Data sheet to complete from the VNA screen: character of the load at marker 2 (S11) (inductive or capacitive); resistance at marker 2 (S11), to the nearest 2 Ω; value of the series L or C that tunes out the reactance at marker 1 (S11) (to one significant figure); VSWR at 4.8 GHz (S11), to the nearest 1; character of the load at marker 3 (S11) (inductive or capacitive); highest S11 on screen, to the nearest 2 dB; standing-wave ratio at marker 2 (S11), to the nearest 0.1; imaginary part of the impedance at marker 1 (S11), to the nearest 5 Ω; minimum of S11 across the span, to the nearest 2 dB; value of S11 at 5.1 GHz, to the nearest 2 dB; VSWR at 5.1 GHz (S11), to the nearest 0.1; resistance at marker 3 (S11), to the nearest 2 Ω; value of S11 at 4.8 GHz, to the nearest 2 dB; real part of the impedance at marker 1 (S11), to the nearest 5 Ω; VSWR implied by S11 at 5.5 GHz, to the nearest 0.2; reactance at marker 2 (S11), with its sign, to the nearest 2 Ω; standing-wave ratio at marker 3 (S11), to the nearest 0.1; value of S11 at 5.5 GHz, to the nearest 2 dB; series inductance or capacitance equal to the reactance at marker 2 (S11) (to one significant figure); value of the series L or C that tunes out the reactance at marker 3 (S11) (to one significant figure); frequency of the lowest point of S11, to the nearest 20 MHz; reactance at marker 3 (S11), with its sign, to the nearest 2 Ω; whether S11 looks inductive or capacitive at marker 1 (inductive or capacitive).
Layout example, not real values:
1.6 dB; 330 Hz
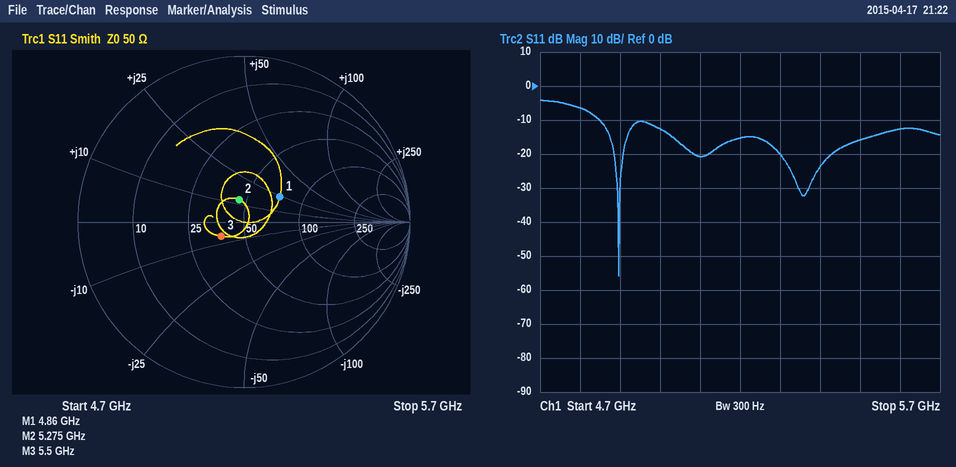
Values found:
inductive; 46 Ω; 1 pF; 3; capacitive; -4 dB; 1.3; +25 Ω; -56 dB; -20 dB; 1.2; 38 Ω; -6 dB; 75 Ω; 1.4; +12 Ω; 1.4; -16 dB; 400 pH; 200 pH; 4.90 GHz; -6 Ω; inductive
